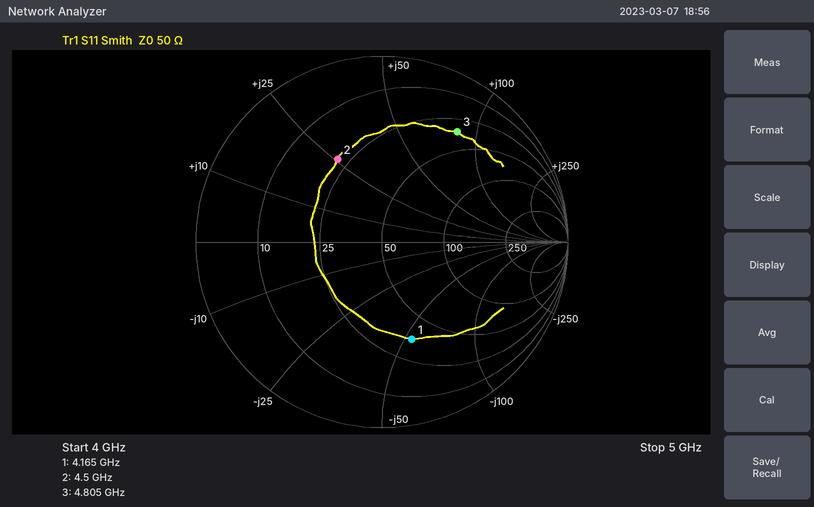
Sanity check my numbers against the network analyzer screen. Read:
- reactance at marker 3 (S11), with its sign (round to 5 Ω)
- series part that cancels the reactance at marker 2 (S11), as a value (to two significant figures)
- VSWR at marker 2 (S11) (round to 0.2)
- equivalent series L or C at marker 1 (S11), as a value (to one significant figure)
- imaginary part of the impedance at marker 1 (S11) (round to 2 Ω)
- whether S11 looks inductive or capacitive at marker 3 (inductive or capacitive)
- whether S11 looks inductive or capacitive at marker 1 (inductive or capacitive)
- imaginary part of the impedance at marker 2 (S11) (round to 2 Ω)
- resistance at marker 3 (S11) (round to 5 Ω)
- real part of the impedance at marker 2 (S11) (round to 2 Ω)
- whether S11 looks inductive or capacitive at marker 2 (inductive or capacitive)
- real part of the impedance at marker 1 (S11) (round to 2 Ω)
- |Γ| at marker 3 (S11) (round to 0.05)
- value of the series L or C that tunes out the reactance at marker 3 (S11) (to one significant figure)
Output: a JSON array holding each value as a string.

["+85 Ω", "1.4 pF", "3.0", "700 fF", "-54 Ω", "inductive", "capacitive", "+26 Ω", "35 Ω", "22 Ω", "inductive", "36 Ω", "0.70", "400 fF"]
